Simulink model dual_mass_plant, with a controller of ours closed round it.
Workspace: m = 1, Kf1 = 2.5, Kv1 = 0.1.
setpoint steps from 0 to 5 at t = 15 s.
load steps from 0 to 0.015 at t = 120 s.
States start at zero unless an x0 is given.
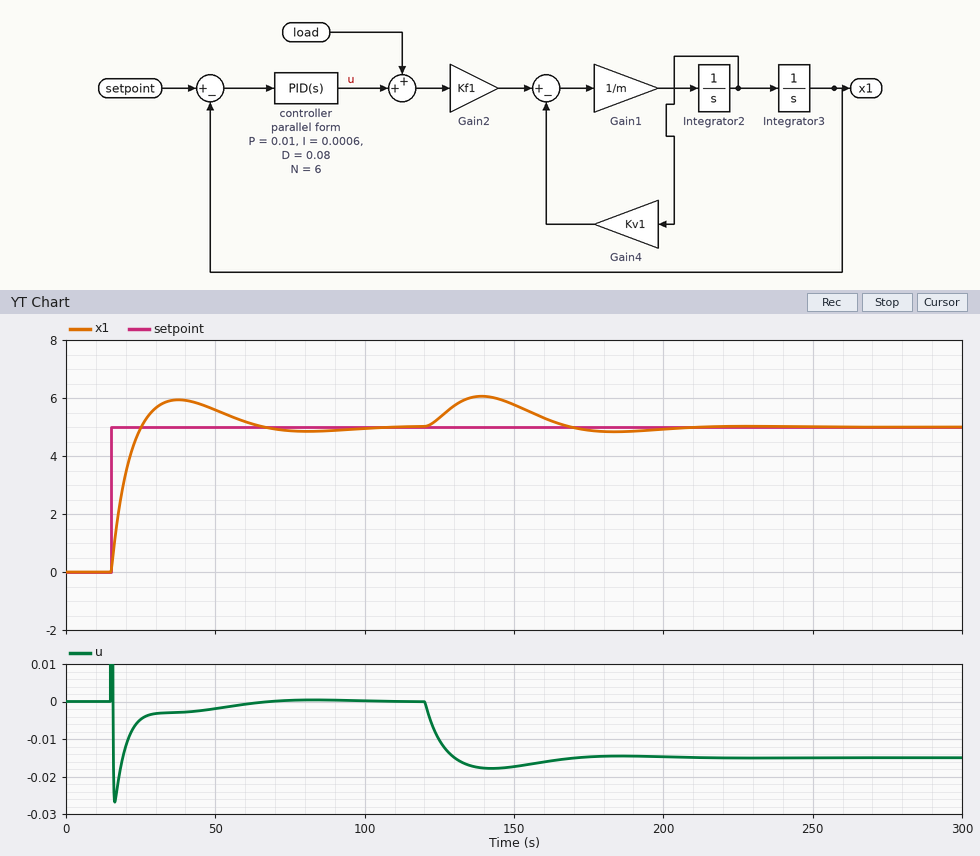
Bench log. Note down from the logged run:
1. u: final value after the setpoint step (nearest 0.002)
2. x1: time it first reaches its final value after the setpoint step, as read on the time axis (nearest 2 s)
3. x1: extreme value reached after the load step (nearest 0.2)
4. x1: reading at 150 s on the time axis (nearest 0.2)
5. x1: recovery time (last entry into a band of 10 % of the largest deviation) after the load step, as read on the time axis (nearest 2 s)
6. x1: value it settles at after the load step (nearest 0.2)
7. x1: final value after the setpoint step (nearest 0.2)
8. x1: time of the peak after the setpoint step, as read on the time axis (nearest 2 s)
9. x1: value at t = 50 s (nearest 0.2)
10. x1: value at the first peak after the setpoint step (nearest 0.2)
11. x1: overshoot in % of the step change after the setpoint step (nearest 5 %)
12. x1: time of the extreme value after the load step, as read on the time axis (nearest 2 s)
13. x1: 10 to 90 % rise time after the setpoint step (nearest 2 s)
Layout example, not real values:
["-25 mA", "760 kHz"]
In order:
["0.000", "26 s", "6.0", "5.8", "196 s", "5.0", "5.0", "38 s", "5.6", "6.0", "20 %", "140 s", "8 s"]
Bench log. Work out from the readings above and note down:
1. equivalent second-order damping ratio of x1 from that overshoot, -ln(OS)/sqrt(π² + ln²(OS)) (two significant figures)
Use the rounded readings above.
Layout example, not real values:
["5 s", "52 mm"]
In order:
["0.46"]
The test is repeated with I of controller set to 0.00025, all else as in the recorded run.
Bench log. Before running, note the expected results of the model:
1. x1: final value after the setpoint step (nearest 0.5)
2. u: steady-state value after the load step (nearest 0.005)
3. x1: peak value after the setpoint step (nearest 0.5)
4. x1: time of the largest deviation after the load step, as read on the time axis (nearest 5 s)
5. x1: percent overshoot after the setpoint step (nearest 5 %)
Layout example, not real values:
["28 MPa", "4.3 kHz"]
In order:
["5.0", "-0.015", "5.5", "145 s", "10 %"]
